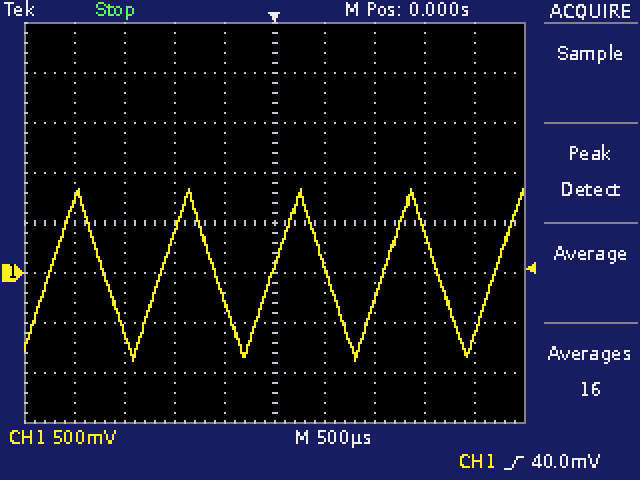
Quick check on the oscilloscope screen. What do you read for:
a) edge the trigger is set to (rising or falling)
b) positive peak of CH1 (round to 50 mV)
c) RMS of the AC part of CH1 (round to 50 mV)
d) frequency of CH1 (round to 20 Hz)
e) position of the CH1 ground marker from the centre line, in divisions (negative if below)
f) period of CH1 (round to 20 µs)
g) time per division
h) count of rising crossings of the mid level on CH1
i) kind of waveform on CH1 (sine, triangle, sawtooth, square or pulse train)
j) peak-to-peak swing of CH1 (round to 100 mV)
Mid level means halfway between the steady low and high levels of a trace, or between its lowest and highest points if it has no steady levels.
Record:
rising
850 mV
500 mV
900 Hz
-1.0 div
1.12 ms
500 µs
5
triangle
1.70 V
